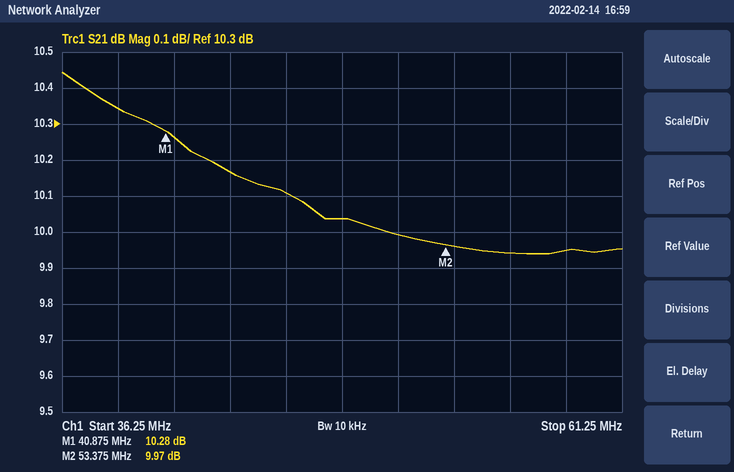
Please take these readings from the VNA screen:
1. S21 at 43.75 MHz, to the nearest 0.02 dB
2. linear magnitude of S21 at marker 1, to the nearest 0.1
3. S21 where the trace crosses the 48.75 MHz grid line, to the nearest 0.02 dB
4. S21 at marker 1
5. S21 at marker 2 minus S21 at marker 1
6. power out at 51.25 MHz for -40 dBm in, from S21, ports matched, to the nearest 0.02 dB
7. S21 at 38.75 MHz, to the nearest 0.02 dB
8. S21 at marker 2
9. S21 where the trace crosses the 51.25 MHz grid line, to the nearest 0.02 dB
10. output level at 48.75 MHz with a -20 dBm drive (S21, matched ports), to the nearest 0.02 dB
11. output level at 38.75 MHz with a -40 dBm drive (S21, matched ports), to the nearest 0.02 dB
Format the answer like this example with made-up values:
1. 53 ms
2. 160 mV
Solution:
1. 10.16 dB
2. 3.3
3. 10.04 dB
4. 10.28 dB
5. -0.31 dB
6. -30.00 dBm
7. 10.34 dB
8. 9.97 dB
9. 10.00 dB
10. -9.96 dBm
11. -29.66 dBm
